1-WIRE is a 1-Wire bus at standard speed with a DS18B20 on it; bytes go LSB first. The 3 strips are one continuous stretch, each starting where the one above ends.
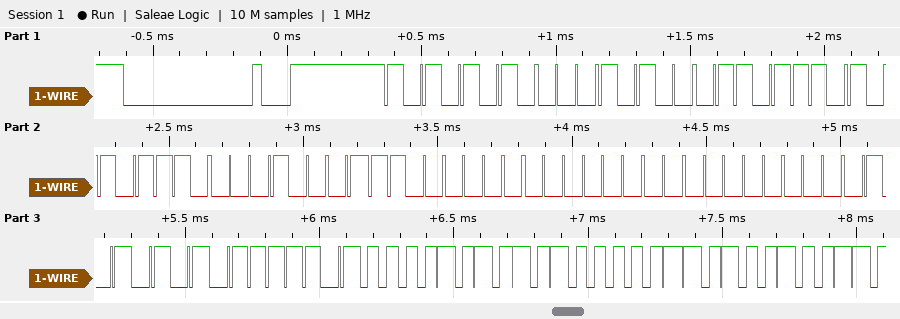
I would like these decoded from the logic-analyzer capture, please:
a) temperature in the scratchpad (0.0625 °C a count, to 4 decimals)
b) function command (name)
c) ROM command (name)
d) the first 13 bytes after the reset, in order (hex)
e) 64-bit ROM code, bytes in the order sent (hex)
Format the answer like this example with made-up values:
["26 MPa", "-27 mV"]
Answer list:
["85.0000 °C", "Read Scratchpad", "Match ROM", "55 28 76 75 88 03 00 00 AA BE 50 05 4B", "28 76 75 88 03 00 00 AA"]
